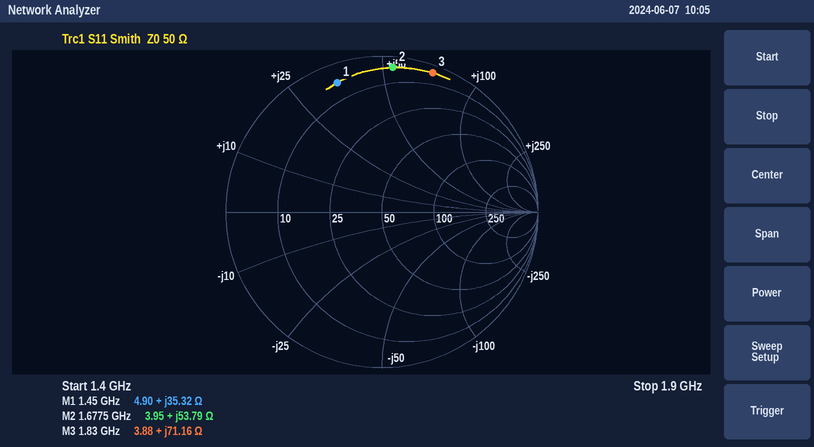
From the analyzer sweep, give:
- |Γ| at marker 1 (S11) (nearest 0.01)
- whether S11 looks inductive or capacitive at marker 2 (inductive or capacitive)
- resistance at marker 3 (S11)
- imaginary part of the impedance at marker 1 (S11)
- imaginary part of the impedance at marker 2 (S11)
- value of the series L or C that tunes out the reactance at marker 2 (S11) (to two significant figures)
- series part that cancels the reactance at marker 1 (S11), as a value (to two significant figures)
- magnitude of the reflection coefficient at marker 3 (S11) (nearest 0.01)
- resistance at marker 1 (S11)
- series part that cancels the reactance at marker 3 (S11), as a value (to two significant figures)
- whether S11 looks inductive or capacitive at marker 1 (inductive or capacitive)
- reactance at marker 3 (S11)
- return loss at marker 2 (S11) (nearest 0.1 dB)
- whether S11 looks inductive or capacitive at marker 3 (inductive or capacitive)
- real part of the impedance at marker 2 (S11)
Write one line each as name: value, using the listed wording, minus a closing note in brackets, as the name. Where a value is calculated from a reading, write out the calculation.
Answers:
|Γ| at marker 1 (S11): 0.88
whether S11 looks inductive or capacitive at marker 2: inductive
resistance at marker 3: 3.88 Ω
imaginary part of the impedance at marker 1: +35.32 Ω
imaginary part of the impedance at marker 2: +53.79 Ω
value of the series L or C that tunes out the reactance at marker 2 (S11): C = 1/(2π × 1.6775 GHz × 53.79 Ω) ≈ 1.8 pF
series part that cancels the reactance at marker 1 (S11), as a value: C = 1/(2π × 1.45 GHz × 35.32 Ω) ≈ 3.1 pF
magnitude of the reflection coefficient at marker 3 (S11): 0.95
resistance at marker 1: 4.90 Ω
series part that cancels the reactance at marker 3 (S11), as a value: C = 1/(2π × 1.83 GHz × 71.16 Ω) ≈ 1.2 pF
whether S11 looks inductive or capacitive at marker 1: inductive
reactance at marker 3: +71.16 Ω
return loss at marker 2 (S11): 0.6 dB
whether S11 looks inductive or capacitive at marker 3: inductive
real part of the impedance at marker 2: 3.95 Ω
